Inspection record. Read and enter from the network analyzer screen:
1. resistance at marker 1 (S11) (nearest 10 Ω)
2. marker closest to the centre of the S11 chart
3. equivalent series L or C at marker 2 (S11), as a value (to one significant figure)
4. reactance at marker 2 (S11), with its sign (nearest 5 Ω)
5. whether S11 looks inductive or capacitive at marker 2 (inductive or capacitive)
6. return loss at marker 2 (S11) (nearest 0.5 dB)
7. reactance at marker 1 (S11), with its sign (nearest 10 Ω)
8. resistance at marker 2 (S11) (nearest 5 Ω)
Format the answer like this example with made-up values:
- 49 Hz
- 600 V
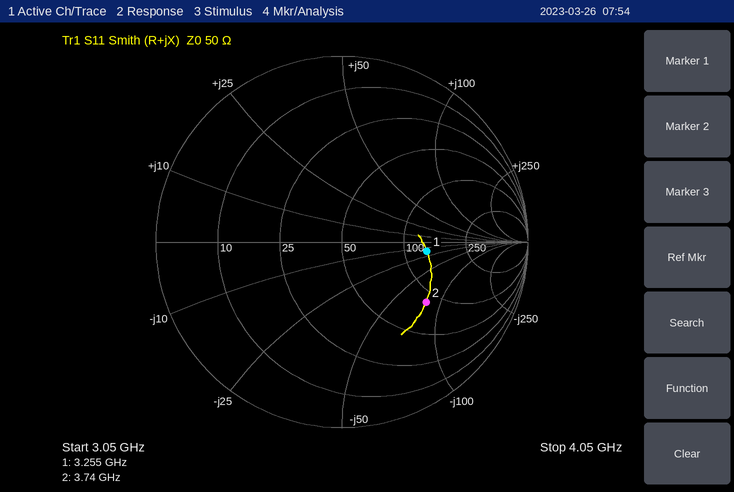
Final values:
- 130 Ω
- marker 1
- 500 fF
- -80 Ω
- capacitive
- 5.0 dB
- -20 Ω
- 85 Ω
